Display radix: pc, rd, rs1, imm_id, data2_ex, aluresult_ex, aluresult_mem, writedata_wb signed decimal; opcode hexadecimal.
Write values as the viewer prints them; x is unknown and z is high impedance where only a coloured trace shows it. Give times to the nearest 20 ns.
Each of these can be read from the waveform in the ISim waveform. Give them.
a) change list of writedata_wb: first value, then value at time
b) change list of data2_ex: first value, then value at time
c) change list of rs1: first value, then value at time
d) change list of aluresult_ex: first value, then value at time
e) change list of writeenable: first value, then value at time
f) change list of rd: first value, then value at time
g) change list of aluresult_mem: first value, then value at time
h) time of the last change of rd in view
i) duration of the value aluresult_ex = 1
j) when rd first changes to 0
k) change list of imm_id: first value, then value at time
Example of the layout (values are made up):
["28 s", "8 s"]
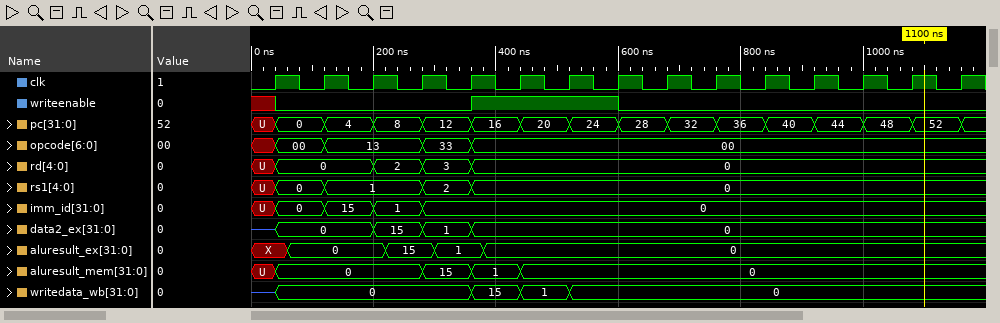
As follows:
["z, 0 at 40 ns, 15 at 360 ns, 1 at 440 ns, 0 at 520 ns", "z, 0 at 40 ns, 15 at 200 ns, 1 at 280 ns, 0 at 360 ns", "U, 0 at 40 ns, 1 at 120 ns, 2 at 280 ns, 0 at 360 ns", "X, 0 at 60 ns, 15 at 220 ns, 1 at 300 ns, 0 at 380 ns", "x, 0 at 40 ns, 1 at 360 ns, 0 at 600 ns", "U, 0 at 40 ns, 2 at 200 ns, 3 at 280 ns, 0 at 360 ns", "U, 0 at 40 ns, 15 at 280 ns, 1 at 360 ns, 0 at 440 ns", "360 ns", "80 ns", "40 ns", "U, 0 at 40 ns, 15 at 120 ns, 1 at 200 ns, 0 at 280 ns"]
